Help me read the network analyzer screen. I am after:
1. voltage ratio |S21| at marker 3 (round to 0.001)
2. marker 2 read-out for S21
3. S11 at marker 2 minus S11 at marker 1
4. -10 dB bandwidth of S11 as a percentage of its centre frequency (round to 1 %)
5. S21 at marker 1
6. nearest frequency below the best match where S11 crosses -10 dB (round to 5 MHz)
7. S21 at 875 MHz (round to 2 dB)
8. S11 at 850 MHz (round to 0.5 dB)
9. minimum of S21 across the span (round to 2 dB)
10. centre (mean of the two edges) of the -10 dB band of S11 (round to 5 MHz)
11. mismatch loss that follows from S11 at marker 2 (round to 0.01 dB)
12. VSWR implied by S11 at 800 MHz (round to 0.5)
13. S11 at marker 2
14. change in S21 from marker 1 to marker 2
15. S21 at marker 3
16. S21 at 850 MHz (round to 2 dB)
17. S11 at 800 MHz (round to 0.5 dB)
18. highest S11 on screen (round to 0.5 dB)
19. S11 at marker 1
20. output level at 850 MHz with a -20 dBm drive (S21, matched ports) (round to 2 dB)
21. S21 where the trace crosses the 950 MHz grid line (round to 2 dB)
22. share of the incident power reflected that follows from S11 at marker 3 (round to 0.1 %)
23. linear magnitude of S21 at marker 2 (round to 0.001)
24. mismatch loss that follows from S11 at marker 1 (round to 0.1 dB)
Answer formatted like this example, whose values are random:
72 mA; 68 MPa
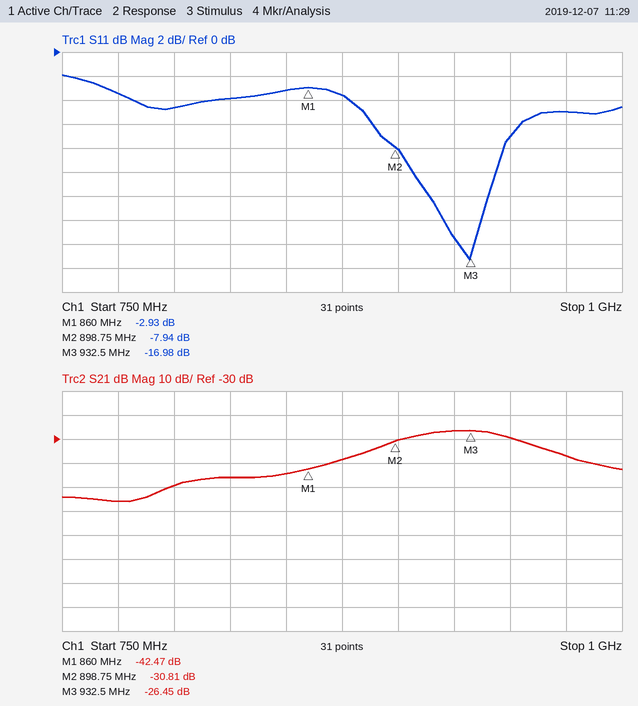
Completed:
0.048; -30.81 dB; -5.01 dB; 4 %; -42.47 dB; 905 MHz; -38 dB; -3.0 dB; -56 dB; 925 MHz; 0.76 dB; 4.0; -7.94 dB; 11.66 dB; -26.45 dB; -44 dB; -4.5 dB; -2.0 dB; -2.93 dB; -64 dBm; -30 dB; 2.0 %; 0.029; 3.1 dB
